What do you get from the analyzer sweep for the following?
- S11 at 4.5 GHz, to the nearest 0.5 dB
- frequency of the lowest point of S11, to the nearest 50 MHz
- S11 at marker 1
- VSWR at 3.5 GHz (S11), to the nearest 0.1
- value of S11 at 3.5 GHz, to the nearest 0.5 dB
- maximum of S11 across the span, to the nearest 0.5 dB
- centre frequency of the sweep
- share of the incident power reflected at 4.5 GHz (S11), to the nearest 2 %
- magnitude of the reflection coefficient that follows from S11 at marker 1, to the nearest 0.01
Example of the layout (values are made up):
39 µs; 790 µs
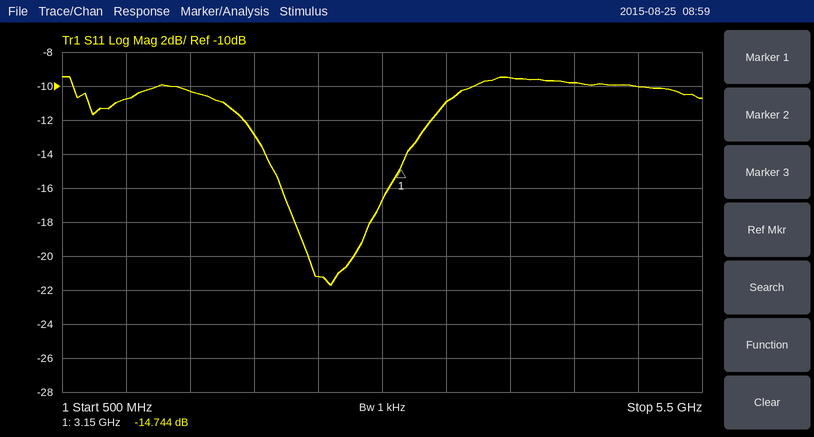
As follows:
-10.0 dB; 2.60 GHz; -14.744 dB; 1.8; -11.0 dB; -9.5 dB; 3 GHz; 10 %; 0.18
